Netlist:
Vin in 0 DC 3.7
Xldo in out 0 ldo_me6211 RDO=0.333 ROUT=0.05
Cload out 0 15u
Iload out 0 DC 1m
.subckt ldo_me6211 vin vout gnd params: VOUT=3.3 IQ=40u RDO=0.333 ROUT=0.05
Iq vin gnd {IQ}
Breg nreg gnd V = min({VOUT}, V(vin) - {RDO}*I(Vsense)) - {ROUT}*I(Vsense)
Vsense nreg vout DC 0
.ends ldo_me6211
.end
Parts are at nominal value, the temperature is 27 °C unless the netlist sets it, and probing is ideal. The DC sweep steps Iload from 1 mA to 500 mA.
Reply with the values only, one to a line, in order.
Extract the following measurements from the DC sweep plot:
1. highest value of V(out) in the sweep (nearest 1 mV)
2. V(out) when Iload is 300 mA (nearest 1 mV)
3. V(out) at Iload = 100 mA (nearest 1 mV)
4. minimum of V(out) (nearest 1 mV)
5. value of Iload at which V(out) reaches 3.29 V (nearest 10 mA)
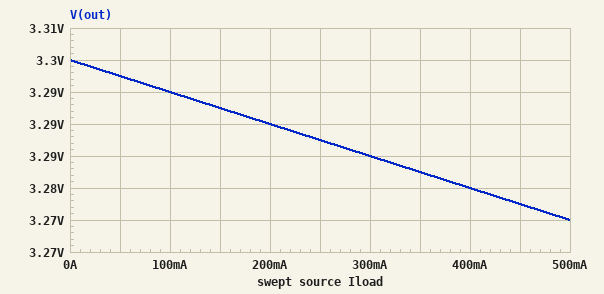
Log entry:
3.300 V
3.285 V
3.295 V
3.275 V
200 mA
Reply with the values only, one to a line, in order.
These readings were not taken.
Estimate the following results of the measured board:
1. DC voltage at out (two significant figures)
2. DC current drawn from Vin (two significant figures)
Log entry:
3.3 V
40 µA
